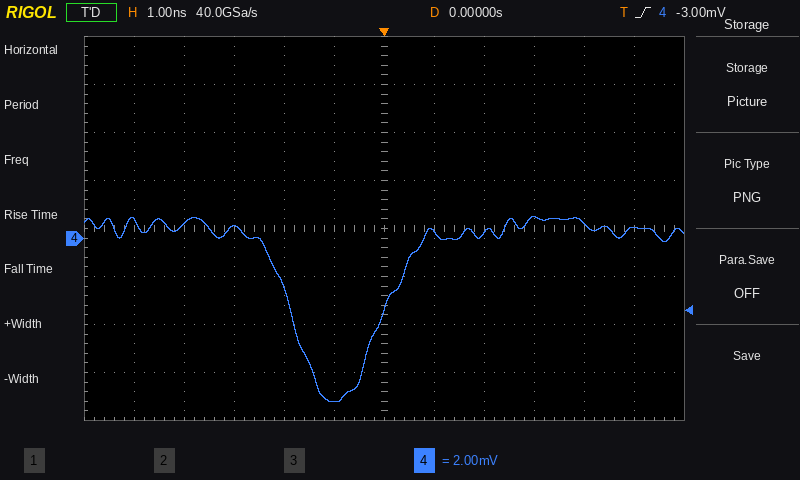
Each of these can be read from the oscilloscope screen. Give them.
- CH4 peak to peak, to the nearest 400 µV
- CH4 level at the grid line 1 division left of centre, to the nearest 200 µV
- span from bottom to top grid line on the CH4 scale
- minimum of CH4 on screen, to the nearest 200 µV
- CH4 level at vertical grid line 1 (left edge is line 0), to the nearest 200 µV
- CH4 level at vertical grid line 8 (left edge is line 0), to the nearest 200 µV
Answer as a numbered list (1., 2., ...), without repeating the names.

1. 7.6 mV
2. -6.8 mV
3. 16 mV
4. -6.8 mV
5. 800 µV
6. 200 µV
